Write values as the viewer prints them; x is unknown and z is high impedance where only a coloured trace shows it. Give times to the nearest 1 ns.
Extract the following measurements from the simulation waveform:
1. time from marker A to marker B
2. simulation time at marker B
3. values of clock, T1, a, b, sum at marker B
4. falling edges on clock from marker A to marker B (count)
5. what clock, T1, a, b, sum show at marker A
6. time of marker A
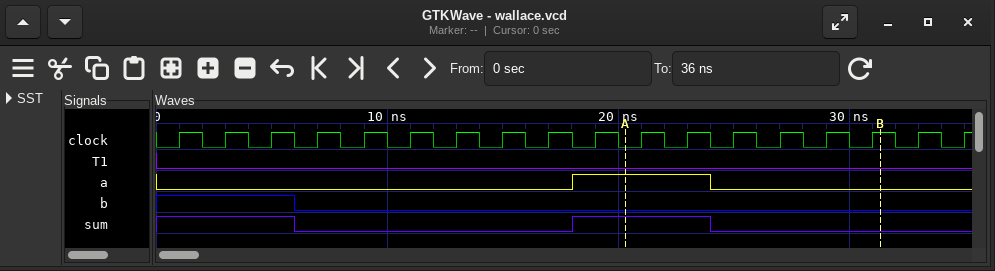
11 ns
31 ns
clock=1, T1=0, a=0, b=0, sum=0
5
clock=0, T1=0, a=1, b=0, sum=1
20 ns
